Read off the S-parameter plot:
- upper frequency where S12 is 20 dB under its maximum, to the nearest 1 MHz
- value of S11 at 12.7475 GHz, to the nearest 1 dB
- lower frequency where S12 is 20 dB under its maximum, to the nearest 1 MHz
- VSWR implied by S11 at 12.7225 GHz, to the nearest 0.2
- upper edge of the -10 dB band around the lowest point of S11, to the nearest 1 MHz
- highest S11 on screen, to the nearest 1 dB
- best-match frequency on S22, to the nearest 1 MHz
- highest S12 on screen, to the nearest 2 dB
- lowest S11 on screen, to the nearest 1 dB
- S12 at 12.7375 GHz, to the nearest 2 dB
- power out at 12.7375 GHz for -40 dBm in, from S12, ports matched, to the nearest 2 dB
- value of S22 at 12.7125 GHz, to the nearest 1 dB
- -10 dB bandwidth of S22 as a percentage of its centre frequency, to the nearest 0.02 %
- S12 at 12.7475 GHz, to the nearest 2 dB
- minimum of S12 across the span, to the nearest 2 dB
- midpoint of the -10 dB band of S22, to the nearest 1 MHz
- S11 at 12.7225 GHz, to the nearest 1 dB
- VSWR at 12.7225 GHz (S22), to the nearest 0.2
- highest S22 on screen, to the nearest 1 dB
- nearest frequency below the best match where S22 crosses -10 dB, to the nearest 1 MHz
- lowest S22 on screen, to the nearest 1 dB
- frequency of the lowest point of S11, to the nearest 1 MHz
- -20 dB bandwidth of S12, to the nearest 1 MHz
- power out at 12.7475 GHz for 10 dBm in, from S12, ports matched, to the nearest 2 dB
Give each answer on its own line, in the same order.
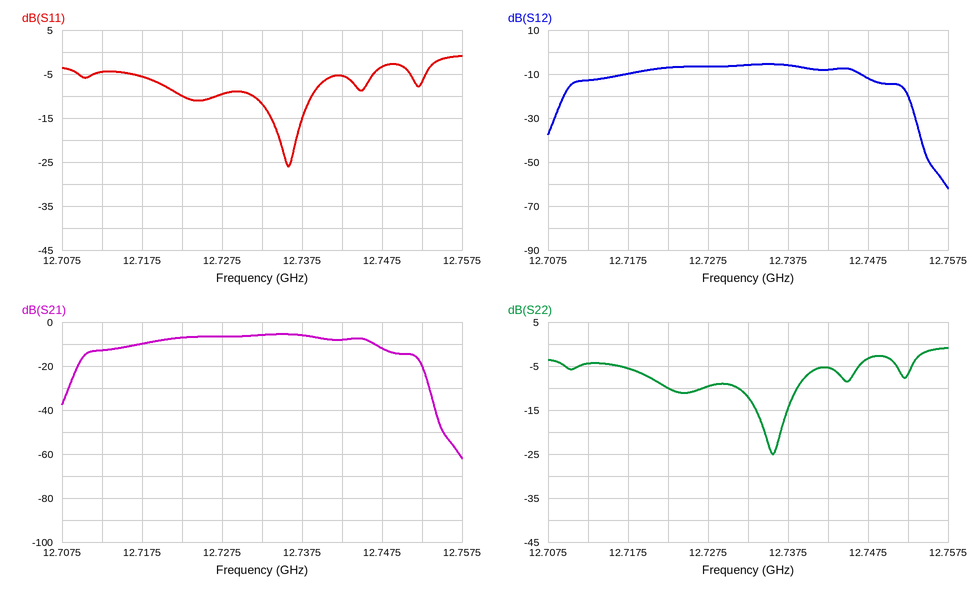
12.753 GHz
-3 dB
12.709 GHz
2.0
12.739 GHz
-1 dB
12.736 GHz
-6 dB
-26 dB
-6 dB
-46 dBm
-4 dB
0.06 %
-12 dB
-62 dB
12.735 GHz
-10 dB
2.0
-1 dB
12.731 GHz
-25 dB
12.736 GHz
44 MHz
-2 dBm
